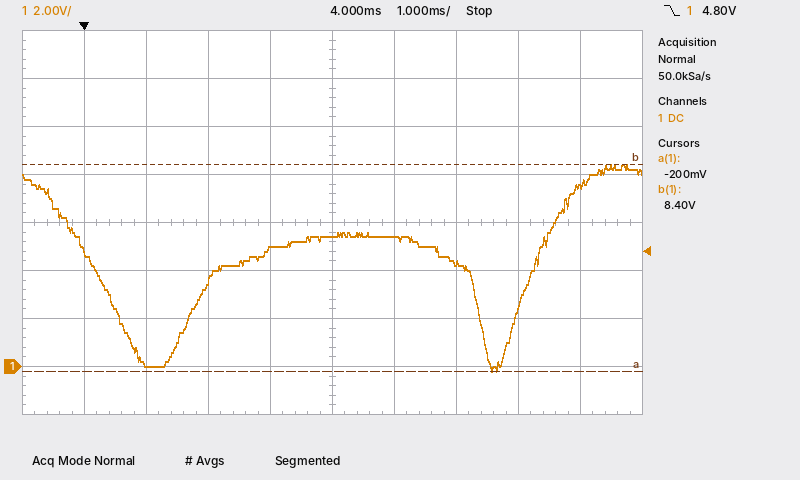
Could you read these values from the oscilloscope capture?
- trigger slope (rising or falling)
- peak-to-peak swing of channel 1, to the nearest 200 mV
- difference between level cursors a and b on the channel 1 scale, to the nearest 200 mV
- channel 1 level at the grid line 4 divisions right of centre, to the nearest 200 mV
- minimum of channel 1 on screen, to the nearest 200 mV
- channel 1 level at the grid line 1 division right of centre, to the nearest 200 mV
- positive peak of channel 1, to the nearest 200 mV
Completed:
falling
8.6 V
8.6 V
7.6 V
-200 mV
5.4 V
8.4 V
